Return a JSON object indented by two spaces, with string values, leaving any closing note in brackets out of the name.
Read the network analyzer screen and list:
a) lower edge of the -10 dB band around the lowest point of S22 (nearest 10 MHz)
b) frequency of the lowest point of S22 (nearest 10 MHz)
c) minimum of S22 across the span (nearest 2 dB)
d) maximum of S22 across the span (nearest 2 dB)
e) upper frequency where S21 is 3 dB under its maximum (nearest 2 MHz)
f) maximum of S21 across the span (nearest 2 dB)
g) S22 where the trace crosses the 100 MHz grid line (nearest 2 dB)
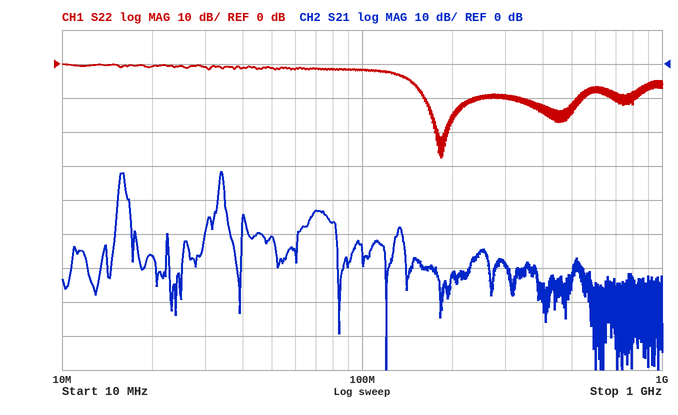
{
  "lower edge of the -10 dB band around the lowest point of S22": "160 MHz",
  "frequency of the lowest point of S22": "180 MHz",
  "minimum of S22 across the span": "-28 dB",
  "maximum of S22 across the span": "0 dB",
  "upper frequency where S21 is 3 dB under its maximum": "34 MHz",
  "maximum of S21 across the span": "-32 dB",
  "S22 where the trace crosses the 100 MHz grid line": "-2 dB"
}
